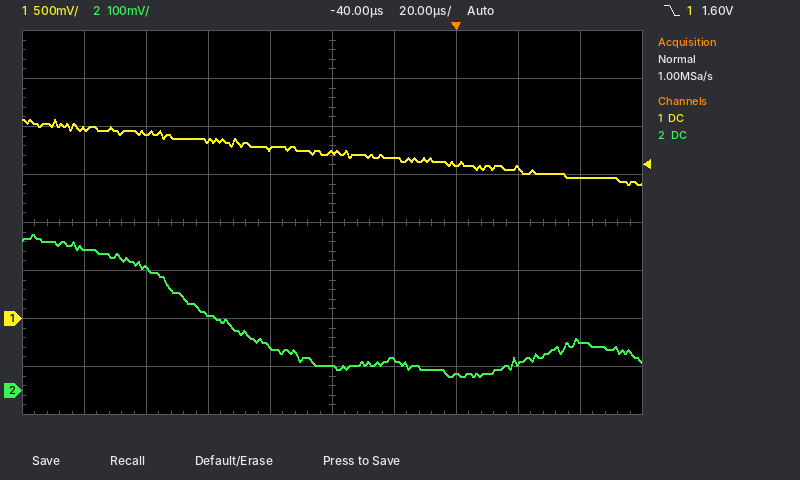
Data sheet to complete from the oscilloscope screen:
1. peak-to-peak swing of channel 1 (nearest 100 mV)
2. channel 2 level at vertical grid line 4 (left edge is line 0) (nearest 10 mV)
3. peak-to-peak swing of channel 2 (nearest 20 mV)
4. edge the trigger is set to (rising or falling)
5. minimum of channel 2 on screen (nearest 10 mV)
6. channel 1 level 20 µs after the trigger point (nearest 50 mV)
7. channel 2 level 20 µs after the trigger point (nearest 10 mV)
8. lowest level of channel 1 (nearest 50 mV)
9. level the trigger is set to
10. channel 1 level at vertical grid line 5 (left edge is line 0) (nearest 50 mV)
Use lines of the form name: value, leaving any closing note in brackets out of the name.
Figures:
peak-to-peak swing of channel 1: 700 mV
channel 2 level at vertical grid line 4 (left edge is line 0): 90 mV
peak-to-peak swing of channel 2: 300 mV
edge the trigger is set to: falling
minimum of channel 2 on screen: 30 mV
channel 1 level 20 µs after the trigger point: 1.55 V
channel 2 level 20 µs after the trigger point: 60 mV
lowest level of channel 1: 1.40 V
level the trigger is set to: 1.60 V
channel 1 level at vertical grid line 5 (left edge is line 0): 1.75 V
